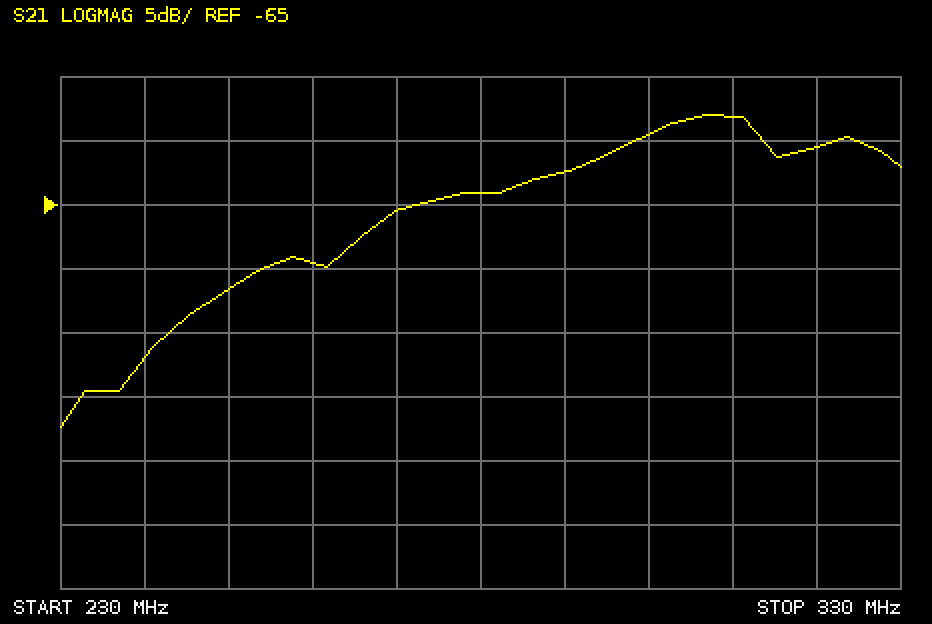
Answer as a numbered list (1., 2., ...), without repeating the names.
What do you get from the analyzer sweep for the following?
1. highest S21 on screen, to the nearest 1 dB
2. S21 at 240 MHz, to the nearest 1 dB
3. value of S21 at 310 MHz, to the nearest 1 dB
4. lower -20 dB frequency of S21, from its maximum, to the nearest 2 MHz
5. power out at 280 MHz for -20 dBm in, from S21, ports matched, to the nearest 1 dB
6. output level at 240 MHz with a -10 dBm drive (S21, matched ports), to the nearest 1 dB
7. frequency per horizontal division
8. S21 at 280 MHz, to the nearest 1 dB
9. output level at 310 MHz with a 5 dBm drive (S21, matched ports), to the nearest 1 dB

1. -58 dB
2. -77 dB
3. -58 dB
4. 238 MHz
5. -84 dBm
6. -87 dBm
7. 10 MHz
8. -64 dB
9. -53 dBm
